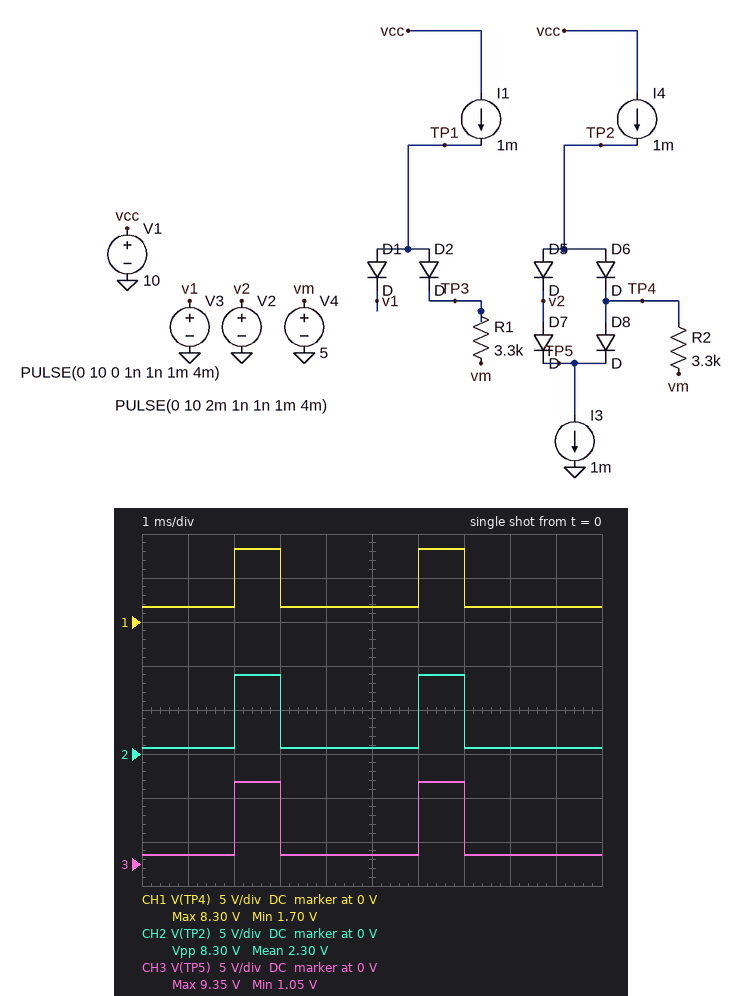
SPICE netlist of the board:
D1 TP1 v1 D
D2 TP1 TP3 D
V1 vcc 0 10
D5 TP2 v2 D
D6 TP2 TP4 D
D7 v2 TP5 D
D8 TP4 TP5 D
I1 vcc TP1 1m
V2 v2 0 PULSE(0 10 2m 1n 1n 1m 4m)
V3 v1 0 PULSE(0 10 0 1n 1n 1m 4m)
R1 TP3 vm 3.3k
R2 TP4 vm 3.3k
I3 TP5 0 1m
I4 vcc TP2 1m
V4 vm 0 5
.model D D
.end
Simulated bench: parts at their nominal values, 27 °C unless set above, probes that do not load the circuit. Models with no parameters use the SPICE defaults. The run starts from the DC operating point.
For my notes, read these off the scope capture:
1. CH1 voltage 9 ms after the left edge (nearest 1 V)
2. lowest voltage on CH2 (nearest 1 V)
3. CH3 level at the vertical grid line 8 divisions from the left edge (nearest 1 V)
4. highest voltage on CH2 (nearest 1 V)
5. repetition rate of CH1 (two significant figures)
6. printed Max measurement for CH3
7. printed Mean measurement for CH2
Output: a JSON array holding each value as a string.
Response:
["2 V", "1 V", "1 V", "9 V", "250 Hz", "9.35 V", "2.30 V"]
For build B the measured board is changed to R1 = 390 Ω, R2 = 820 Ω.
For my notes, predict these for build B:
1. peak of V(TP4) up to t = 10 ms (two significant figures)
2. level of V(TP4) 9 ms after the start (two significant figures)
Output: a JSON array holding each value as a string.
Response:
["5.8 V", "4.2 V"]
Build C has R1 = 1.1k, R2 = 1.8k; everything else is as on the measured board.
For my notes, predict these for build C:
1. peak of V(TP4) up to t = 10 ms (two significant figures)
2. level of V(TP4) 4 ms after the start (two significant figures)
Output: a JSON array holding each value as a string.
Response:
["6.8 V", "3.2 V"]
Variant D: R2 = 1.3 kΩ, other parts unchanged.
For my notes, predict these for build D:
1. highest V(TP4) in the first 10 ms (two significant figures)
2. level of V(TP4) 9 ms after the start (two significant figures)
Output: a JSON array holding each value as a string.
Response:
["6.3 V", "3.7 V"]
